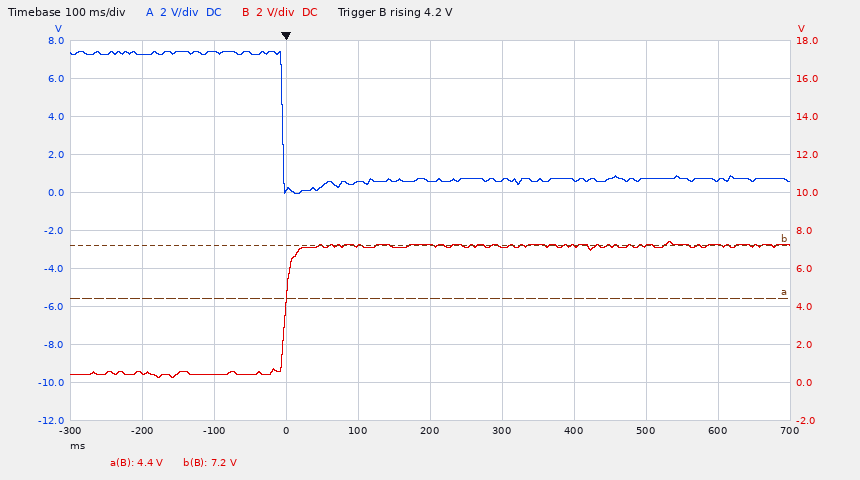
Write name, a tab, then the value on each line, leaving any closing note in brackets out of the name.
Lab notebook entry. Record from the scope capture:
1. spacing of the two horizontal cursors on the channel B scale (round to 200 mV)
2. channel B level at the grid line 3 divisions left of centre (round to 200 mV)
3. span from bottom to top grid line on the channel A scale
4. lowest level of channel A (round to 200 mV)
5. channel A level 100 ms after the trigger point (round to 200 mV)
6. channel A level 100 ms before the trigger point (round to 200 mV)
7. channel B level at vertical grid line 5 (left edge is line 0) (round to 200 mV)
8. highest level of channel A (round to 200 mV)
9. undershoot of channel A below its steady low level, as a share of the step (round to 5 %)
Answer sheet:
spacing of the two horizontal cursors on the channel B scale	2.8 V
channel B level at the grid line 3 divisions left of centre	400 mV
span from bottom to top grid line on the channel A scale	20 V
lowest level of channel A	0.0 V
channel A level 100 ms after the trigger point	600 mV
channel A level 100 ms before the trigger point	7.4 V
channel B level at vertical grid line 5 (left edge is line 0)	7.2 V
highest level of channel A	7.4 V
undershoot of channel A below its steady low level, as a share of the step	10 %
